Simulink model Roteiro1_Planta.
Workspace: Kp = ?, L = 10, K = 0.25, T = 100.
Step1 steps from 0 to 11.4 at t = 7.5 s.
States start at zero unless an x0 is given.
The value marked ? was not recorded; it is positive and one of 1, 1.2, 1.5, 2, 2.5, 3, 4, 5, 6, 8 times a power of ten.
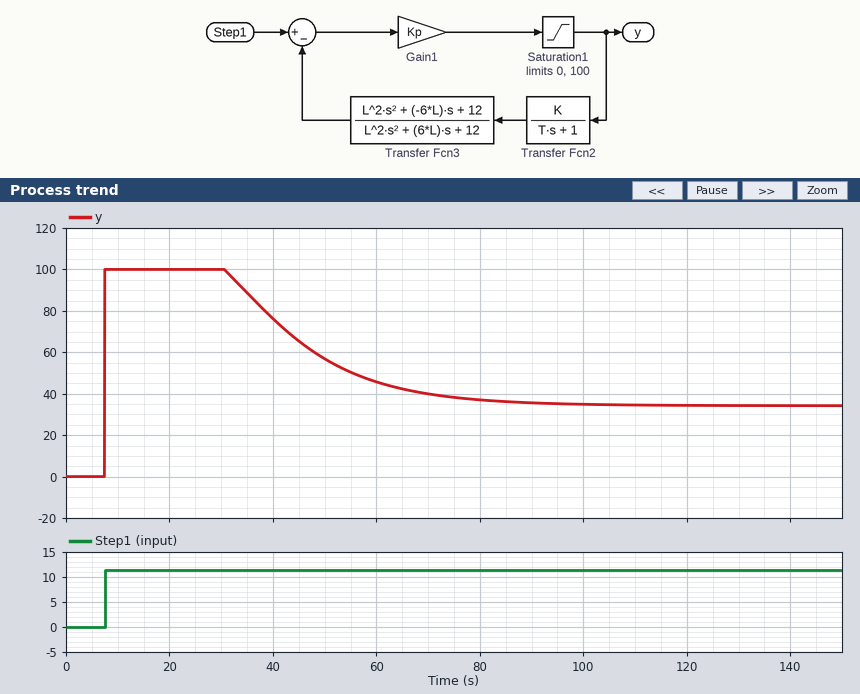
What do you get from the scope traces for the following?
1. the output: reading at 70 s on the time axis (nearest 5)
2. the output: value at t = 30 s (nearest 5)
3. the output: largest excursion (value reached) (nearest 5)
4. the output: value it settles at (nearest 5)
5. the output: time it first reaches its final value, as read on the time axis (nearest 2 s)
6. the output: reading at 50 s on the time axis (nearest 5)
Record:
40
100
100
35
8 s
55
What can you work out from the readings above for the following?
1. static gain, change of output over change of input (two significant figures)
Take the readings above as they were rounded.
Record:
3.1
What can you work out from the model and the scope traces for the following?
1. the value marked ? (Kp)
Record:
12
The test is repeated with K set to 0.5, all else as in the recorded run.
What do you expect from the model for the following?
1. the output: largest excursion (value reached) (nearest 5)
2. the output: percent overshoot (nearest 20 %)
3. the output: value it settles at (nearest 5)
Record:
100
420 %
20
